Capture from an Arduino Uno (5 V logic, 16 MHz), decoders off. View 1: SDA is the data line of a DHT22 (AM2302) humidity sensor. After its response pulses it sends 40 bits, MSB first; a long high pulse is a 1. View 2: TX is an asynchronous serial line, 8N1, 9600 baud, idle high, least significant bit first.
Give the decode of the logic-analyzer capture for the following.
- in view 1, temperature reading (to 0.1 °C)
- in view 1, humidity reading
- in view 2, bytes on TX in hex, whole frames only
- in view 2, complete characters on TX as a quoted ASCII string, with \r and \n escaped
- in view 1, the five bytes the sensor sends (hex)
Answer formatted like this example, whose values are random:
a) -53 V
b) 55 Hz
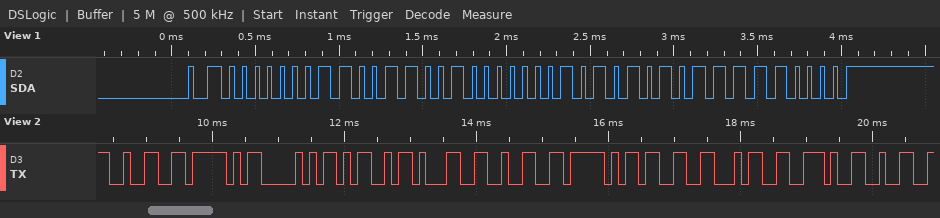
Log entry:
a) 34.1 °C
b) 40.9 %
c) 32 5F 50 4D 31 32 5F 33 34 2E 32
d) "2_PM12_34.2"
e) 01 99 01 55 F0
